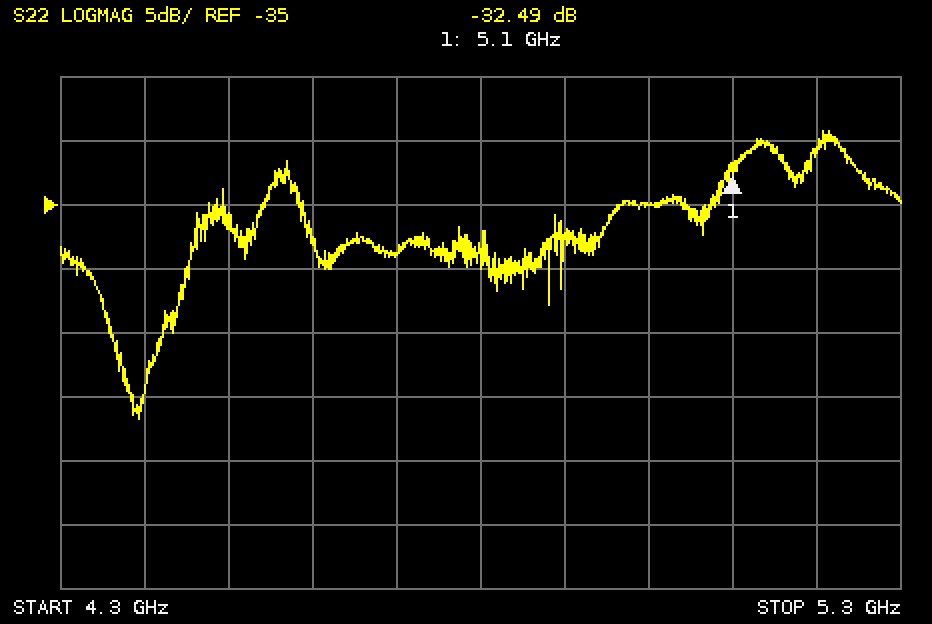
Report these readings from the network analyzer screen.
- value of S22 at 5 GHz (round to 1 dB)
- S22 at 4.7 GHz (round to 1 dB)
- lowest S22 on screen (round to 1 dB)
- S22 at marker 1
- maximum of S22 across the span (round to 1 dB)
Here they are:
-35 dB
-39 dB
-52 dB
-32.49 dB
-29 dB
